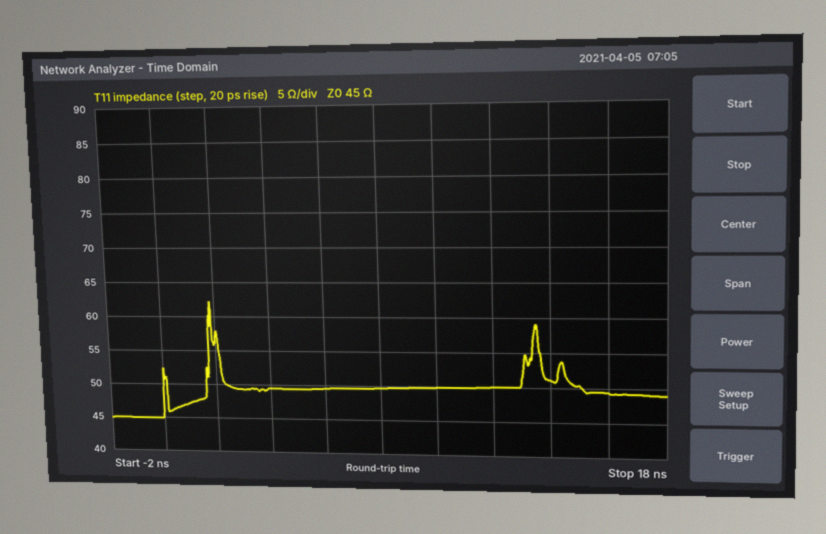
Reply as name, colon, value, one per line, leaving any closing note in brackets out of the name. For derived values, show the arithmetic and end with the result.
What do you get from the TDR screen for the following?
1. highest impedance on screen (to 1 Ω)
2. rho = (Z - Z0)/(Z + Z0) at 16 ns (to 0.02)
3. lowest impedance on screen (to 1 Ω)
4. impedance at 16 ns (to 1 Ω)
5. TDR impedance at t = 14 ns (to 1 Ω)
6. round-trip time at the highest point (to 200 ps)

highest impedance on screen: 62 Ω
rho = (Z - Z0)/(Z + Z0) at 16 ns: (49 − 45)/(49 + 45) ≈ +0.04
lowest impedance on screen: 45 Ω
impedance at 16 ns: 49 Ω
TDR impedance at t = 14 ns: 51 Ω
round-trip time at the highest point: 1.8 ns
